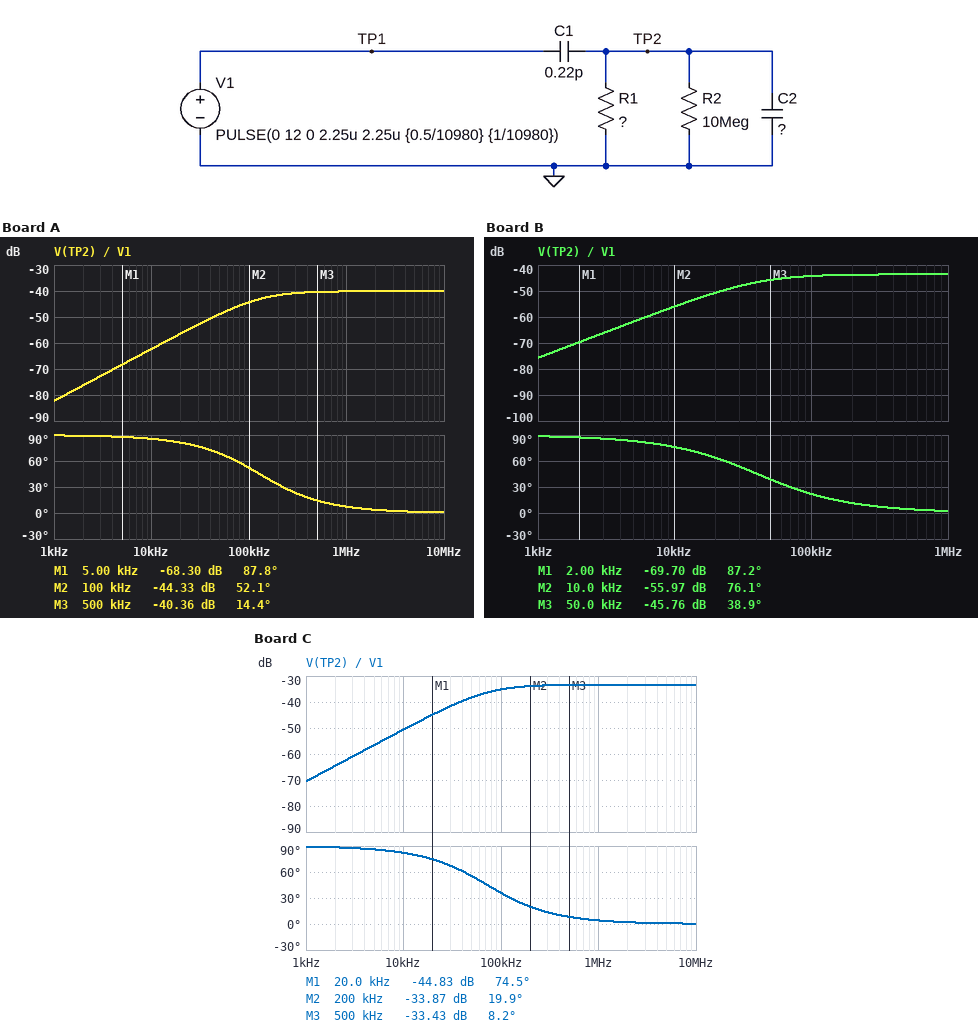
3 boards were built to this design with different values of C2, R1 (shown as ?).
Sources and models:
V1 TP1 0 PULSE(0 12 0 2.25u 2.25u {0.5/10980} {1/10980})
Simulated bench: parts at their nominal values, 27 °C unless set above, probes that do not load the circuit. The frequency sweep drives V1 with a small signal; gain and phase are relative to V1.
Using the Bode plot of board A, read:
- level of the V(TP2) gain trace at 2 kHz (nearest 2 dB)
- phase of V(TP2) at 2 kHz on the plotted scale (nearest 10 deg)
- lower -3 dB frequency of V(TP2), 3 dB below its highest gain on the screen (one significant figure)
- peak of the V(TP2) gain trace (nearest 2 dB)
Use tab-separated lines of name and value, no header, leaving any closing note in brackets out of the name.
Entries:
level of the V(TP2) gain trace at 2 kHz	-76 dB
phase of V(TP2) at 2 kHz on the plotted scale	90 deg
lower -3 dB frequency of V(TP2), 3 dB below its highest gain on the screen	100 kHz
peak of the V(TP2) gain trace	-40 dB
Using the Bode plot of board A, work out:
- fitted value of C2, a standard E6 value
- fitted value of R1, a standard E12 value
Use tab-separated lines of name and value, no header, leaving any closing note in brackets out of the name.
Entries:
fitted value of C2, a standard E6 value	22 pF
fitted value of R1, a standard E12 value	56 kΩ
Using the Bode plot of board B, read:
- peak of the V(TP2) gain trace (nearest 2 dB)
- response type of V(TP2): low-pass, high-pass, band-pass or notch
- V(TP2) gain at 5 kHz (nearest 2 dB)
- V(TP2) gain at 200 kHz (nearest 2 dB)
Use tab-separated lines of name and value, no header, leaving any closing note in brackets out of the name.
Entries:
peak of the V(TP2) gain trace	-44 dB
response type of V(TP2): low-pass, high-pass, band-pass or notch	high-pass
V(TP2) gain at 5 kHz	-62 dB
V(TP2) gain at 200 kHz	-44 dB
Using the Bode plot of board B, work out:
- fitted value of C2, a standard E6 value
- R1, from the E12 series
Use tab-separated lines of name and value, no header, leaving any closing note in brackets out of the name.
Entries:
fitted value of C2, a standard E6 value	33 pF
R1, from the E12 series	120 kΩ
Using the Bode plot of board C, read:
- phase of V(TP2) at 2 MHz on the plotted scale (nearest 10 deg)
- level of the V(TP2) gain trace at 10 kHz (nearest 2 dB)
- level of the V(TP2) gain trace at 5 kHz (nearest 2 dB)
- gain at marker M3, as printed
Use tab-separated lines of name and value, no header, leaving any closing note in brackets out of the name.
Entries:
phase of V(TP2) at 2 MHz on the plotted scale	0 deg
level of the V(TP2) gain trace at 10 kHz	-50 dB
level of the V(TP2) gain trace at 5 kHz	-56 dB
gain at marker M3, as printed	-33.43 dB
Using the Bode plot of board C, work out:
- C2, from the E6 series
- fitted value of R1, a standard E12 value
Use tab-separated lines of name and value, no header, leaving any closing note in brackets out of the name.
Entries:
C2, from the E6 series	10 pF
fitted value of R1, a standard E12 value	220 kΩ
